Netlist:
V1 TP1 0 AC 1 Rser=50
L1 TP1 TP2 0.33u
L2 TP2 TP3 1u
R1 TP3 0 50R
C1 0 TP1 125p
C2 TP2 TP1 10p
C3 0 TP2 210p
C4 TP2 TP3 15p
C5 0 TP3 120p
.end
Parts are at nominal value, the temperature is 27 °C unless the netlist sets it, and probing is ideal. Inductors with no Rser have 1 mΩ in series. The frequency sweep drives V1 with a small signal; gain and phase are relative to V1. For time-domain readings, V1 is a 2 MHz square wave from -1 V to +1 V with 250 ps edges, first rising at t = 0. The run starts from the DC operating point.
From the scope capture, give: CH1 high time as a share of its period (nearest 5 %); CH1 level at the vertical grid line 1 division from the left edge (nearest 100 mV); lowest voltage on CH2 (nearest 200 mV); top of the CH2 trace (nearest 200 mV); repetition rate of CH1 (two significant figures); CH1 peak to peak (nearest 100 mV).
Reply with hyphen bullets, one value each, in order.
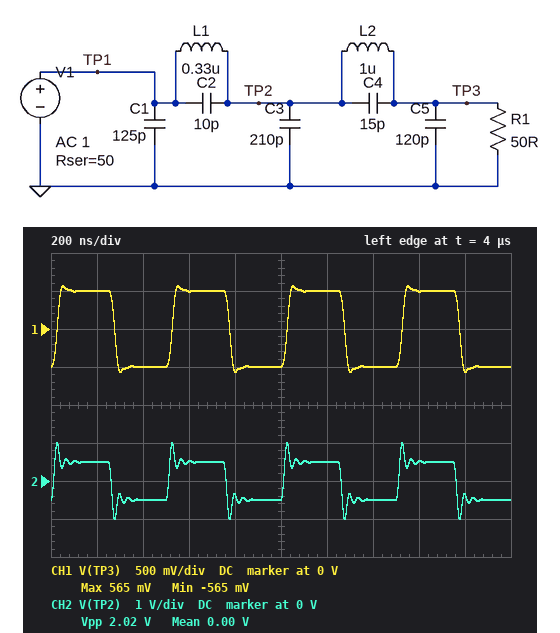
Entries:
- 50 %
- 500 mV
- -1.0 V
- 1.0 V
- 2.0 MHz
- 1.1 V
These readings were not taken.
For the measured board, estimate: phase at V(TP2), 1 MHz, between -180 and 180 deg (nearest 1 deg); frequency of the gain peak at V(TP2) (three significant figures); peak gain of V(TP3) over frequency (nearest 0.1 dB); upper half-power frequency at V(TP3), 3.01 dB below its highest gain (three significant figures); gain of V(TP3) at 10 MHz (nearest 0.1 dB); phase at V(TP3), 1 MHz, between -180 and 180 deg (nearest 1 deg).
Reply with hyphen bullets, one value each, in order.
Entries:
- -2 deg
- 24.6 MHz
- -6.0 dB
- 14.8 MHz
- -6.8 dB
- -9 deg
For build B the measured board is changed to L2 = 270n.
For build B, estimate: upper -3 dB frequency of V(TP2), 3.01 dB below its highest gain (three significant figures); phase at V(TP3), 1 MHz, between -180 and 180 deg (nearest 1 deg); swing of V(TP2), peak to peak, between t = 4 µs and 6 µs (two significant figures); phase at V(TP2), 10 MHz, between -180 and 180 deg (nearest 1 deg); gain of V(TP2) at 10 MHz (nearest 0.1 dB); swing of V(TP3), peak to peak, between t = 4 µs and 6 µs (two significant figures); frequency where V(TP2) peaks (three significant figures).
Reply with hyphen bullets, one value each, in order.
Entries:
- 35.9 MHz
- -6 deg
- 1.2 V
- -40 deg
- -6.8 dB
- 1.3 V
- 32.1 MHz
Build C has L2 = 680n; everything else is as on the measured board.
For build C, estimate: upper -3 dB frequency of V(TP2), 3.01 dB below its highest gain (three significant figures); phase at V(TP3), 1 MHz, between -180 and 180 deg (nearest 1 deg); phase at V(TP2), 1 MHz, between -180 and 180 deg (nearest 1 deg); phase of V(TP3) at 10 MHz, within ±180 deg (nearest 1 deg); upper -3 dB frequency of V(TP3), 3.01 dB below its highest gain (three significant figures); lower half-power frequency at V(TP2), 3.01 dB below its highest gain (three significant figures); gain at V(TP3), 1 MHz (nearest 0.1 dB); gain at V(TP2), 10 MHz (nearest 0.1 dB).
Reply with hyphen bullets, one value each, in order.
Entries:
- 30.1 MHz
- -8 deg
- -3 deg
- -81 deg
- 21.0 MHz
- 17.0 MHz
- -6.0 dB
- -5.2 dB
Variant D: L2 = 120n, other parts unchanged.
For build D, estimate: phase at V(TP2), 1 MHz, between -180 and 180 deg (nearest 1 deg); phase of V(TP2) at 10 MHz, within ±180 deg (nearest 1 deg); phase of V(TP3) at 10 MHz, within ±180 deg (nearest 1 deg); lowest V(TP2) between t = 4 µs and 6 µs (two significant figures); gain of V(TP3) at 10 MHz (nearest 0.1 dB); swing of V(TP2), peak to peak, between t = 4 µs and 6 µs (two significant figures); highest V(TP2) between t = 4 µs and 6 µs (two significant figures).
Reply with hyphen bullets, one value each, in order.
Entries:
- -5 deg
- -46 deg
- -55 deg
- -510 mV
- -6.5 dB
- 1.0 V
- 510 mV
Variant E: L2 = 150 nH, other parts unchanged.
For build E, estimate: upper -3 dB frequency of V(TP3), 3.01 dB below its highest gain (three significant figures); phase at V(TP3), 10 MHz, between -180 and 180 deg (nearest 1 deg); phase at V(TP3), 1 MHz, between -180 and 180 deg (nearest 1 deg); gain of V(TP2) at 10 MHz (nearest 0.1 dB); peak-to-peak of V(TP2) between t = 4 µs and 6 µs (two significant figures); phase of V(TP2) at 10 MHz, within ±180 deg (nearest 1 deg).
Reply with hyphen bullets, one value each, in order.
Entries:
- 30.5 MHz
- -56 deg
- -6 deg
- -6.9 dB
- 1.0 V
- -45 deg
